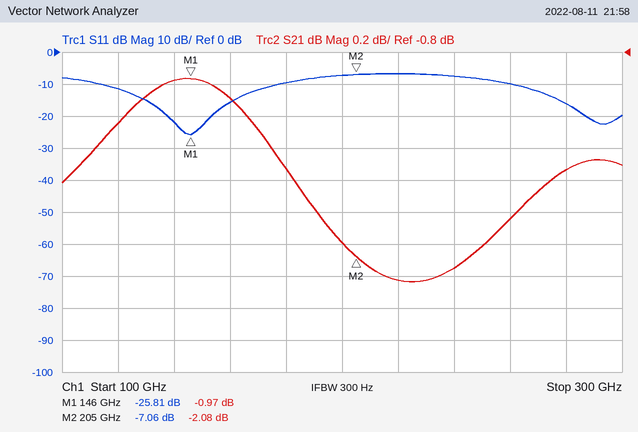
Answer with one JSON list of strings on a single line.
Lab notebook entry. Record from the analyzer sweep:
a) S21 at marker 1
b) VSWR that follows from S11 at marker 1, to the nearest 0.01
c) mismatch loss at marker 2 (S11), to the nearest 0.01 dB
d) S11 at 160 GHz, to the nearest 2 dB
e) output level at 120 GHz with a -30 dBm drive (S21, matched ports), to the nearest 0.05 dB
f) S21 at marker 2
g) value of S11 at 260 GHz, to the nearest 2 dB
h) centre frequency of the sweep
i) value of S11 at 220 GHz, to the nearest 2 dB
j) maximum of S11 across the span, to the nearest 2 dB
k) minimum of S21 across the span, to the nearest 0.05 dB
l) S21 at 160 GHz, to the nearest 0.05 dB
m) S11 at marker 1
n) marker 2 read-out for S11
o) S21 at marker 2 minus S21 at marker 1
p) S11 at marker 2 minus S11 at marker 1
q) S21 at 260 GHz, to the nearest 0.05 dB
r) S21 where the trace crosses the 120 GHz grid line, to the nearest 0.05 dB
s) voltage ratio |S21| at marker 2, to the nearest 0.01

["-0.97 dB", "1.11", "0.95 dB", "-16 dB", "-31.25 dBm", "-2.08 dB", "-10 dB", "200 GHz", "-6 dB", "-6 dB", "-2.25 dB", "-1.10 dB", "-25.81 dB", "-7.06 dB", "-1.11 dB", "18.75 dB", "-1.85 dB", "-1.25 dB", "0.79"]
